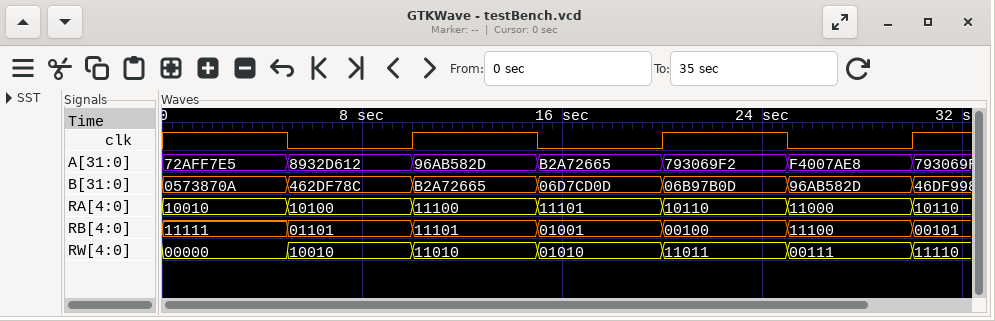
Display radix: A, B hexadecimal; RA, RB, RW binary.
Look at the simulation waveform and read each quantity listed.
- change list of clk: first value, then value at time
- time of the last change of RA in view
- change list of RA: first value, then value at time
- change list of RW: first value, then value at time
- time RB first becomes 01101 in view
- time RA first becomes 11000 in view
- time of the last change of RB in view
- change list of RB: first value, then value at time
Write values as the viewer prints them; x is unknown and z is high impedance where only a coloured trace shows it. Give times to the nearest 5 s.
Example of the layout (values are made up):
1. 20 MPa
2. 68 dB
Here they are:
1. 1, 0 at 5 s, 1 at 10 s, 0 at 15 s, 1 at 20 s, 0 at 25 s, 1 at 30 s
2. 30 s
3. 10010, 10100 at 5 s, 11100 at 10 s, 11101 at 15 s, 10110 at 20 s, 11000 at 25 s, 10110 at 30 s
4. 00000, 10010 at 5 s, 11010 at 10 s, 01010 at 15 s, 11011 at 20 s, 00111 at 25 s, 11110 at 30 s
5. 5 s
6. 25 s
7. 30 s
8. 11111, 01101 at 5 s, 11101 at 10 s, 01001 at 15 s, 00100 at 20 s, 11100 at 25 s, 00101 at 30 s
